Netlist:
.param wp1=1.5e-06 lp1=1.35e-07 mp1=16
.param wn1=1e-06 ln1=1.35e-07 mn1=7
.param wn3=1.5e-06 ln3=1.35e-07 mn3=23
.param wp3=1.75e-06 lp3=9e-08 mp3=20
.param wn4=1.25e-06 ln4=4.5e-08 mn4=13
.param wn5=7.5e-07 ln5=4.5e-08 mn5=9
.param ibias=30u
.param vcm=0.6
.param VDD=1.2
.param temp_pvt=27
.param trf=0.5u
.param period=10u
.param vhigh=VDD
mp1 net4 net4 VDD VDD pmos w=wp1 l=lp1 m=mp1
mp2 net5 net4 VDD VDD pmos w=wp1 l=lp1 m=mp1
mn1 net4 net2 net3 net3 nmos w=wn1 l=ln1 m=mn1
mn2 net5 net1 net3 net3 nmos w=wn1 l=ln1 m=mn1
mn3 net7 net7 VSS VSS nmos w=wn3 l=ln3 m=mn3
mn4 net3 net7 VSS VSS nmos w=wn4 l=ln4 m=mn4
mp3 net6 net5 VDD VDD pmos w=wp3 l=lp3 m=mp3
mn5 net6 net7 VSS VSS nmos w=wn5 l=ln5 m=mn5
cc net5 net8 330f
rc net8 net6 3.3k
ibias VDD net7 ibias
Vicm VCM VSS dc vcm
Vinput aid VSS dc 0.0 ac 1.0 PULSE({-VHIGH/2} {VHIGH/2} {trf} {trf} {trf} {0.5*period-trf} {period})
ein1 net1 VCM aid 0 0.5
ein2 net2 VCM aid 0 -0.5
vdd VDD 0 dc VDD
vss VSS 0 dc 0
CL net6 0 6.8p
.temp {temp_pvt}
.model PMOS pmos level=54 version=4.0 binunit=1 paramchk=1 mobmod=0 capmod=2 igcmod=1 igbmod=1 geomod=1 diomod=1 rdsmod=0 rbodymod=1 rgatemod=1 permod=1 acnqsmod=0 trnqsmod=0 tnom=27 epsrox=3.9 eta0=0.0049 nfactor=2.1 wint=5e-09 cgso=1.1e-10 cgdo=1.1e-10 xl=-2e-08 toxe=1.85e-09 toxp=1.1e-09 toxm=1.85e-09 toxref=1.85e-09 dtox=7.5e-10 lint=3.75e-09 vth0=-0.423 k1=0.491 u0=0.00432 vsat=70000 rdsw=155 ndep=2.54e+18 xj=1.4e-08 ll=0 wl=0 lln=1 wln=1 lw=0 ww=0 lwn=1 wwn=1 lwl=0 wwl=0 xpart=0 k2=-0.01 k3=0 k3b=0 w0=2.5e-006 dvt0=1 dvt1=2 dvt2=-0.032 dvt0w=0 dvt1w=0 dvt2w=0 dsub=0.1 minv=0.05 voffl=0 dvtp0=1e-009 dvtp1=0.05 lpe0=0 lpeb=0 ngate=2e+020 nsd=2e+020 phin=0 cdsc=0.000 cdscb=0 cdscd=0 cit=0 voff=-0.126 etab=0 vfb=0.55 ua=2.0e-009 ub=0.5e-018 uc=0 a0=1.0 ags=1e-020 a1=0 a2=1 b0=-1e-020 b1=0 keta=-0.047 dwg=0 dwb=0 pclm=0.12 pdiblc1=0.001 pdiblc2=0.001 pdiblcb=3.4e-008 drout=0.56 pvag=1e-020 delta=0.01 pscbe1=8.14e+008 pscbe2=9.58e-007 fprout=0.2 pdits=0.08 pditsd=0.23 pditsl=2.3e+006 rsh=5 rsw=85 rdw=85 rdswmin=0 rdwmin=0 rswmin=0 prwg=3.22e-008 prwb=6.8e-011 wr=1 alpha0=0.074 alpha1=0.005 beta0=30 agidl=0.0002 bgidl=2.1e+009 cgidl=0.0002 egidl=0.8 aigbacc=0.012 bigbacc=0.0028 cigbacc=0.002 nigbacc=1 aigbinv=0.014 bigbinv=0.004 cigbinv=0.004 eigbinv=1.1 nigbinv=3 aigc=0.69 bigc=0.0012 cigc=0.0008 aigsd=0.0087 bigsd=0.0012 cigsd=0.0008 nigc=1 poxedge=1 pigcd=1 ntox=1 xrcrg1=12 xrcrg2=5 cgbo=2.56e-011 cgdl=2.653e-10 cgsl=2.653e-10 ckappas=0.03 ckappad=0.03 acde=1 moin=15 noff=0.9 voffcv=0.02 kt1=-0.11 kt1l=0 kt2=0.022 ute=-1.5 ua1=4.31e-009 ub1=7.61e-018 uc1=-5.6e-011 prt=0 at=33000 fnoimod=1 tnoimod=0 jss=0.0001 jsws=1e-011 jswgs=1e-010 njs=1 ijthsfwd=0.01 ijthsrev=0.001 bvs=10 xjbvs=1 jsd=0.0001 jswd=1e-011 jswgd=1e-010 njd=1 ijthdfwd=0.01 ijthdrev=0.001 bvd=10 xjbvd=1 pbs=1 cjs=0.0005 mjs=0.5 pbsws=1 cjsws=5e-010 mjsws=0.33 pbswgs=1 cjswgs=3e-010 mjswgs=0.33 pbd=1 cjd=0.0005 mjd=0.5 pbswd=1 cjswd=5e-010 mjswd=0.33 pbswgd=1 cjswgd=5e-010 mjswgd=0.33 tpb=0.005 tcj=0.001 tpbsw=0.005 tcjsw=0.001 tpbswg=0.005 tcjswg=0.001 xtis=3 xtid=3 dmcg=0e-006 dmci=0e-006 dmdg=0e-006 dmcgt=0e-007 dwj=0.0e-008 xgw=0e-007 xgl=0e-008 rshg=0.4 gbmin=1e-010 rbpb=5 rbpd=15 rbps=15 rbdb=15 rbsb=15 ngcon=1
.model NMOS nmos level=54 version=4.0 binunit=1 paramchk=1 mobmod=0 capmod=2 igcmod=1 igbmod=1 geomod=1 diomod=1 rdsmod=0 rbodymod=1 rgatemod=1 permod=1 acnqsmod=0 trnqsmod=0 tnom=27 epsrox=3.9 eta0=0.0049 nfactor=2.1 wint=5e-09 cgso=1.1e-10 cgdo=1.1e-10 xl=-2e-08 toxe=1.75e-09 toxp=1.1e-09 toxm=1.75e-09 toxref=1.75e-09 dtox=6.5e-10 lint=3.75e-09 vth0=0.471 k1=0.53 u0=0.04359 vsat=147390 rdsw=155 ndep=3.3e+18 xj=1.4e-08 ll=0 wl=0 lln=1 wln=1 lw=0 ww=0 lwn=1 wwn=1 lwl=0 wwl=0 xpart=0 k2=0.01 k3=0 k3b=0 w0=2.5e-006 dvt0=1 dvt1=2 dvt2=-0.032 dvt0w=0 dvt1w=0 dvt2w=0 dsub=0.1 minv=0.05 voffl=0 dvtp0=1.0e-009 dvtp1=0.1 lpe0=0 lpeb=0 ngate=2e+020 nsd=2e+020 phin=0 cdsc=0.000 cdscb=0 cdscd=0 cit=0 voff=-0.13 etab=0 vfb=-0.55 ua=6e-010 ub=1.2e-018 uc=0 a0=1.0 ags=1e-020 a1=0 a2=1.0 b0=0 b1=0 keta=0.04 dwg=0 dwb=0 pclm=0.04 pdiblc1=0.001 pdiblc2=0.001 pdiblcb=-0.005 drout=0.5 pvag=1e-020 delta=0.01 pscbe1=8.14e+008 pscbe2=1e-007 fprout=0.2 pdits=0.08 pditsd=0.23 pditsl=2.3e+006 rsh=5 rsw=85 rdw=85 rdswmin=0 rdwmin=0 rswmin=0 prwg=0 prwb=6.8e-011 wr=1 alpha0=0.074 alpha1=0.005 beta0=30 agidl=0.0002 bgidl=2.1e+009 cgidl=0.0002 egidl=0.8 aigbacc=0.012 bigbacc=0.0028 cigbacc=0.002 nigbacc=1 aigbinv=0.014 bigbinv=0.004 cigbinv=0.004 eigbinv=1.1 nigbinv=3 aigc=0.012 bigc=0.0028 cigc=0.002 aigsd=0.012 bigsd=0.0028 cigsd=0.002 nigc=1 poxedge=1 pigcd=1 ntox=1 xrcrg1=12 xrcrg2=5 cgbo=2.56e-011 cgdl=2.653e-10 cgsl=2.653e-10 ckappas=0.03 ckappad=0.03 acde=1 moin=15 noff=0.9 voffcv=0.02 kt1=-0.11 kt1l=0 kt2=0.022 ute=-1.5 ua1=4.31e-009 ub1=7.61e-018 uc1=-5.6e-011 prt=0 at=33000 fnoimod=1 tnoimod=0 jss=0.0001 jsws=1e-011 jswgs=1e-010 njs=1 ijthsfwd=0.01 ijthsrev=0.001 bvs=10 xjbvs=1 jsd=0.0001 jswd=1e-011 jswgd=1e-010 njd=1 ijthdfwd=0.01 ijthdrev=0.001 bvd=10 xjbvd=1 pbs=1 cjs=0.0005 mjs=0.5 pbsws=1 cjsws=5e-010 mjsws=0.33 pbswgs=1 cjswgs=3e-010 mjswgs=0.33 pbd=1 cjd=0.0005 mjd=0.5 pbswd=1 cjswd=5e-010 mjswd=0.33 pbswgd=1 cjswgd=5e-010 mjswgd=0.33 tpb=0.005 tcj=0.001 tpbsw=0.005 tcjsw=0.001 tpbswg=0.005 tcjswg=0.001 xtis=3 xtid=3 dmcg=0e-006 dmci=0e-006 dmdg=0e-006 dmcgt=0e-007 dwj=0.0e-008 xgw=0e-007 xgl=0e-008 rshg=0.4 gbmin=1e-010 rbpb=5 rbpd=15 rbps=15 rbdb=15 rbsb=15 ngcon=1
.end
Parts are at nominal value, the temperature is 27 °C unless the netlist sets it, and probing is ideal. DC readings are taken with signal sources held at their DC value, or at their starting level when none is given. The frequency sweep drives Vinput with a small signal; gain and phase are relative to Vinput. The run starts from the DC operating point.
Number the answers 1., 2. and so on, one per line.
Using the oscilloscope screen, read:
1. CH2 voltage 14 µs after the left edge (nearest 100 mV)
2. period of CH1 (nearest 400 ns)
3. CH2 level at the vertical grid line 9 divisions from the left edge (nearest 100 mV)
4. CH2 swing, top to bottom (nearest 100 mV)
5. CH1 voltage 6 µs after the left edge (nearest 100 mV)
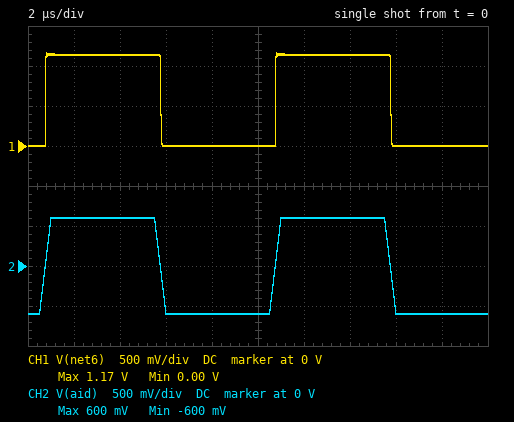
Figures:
1. 600 mV
2. 10.0 µs
3. -600 mV
4. 1.2 V
5. 0 V
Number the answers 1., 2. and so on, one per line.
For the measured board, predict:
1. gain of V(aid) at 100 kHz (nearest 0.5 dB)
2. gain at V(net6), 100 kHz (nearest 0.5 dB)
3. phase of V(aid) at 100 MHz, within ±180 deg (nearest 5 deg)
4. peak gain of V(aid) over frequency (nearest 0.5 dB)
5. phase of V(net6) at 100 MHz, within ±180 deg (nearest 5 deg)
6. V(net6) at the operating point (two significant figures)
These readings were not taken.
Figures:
1. 0 dB
2. 48.5 dB
3. 0 deg
4. 0 dB
5. -130 deg
6. 520 mV
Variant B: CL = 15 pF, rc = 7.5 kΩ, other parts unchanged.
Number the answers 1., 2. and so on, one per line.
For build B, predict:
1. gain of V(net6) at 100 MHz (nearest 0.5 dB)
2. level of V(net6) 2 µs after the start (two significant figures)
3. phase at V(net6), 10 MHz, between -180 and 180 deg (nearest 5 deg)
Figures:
1. 3.5 dB
2. 1.1 V
3. -95 deg
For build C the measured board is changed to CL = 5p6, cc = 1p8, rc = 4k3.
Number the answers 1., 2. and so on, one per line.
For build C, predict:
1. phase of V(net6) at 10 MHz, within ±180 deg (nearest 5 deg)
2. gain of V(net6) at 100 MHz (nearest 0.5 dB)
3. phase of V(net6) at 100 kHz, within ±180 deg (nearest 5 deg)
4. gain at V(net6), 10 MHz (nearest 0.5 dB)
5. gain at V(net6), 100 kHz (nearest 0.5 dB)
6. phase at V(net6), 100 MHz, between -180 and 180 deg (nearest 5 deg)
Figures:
1. -75 deg
2. 6.0 dB
3. -20 deg
4. 17.5 dB
5. 48.0 dB
6. -80 deg
